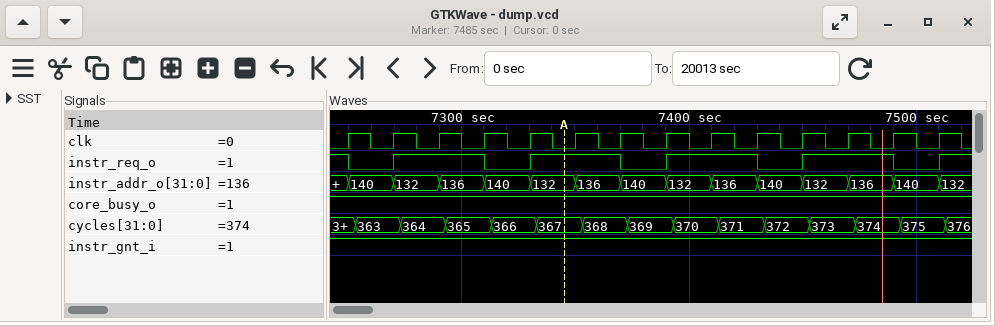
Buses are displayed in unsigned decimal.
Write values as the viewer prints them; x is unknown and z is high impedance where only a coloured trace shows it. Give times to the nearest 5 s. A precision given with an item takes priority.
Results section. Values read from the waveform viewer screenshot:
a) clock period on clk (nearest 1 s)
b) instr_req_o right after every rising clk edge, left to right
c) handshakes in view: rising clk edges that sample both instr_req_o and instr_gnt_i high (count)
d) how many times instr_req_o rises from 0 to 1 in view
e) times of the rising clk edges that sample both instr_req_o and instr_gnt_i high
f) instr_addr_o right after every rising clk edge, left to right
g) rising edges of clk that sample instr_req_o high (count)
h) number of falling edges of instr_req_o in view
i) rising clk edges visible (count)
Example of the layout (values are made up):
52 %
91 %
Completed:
20 s
0 1 1 0 1 1 0 1 1 0 1 1 0 1
9
5
7250 s, 7290 s, 7310 s, 7350 s, 7370 s, 7410 s, 7430 s, 7470 s, 7490 s
140, 132, 136, 140, 132, 136, 140, 132, 136, 140, 132, 136, 140, 132
9
5
14
